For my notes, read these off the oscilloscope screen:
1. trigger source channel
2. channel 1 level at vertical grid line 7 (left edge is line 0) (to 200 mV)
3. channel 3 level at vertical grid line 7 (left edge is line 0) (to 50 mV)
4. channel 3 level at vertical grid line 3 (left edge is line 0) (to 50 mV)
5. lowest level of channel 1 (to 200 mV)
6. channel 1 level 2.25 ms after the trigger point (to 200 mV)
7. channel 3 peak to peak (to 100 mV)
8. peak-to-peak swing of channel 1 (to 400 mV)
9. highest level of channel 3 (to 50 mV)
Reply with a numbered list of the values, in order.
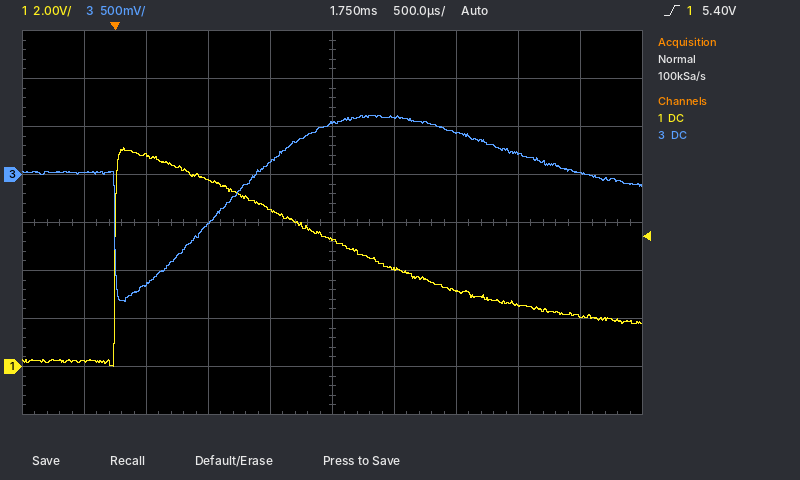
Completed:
1. channel 1
2. 3.2 V
3. 450 mV
4. -500 mV
5. 0.0 V
6. 4.0 V
7. 1.90 V
8. 9.2 V
9. 600 mV
